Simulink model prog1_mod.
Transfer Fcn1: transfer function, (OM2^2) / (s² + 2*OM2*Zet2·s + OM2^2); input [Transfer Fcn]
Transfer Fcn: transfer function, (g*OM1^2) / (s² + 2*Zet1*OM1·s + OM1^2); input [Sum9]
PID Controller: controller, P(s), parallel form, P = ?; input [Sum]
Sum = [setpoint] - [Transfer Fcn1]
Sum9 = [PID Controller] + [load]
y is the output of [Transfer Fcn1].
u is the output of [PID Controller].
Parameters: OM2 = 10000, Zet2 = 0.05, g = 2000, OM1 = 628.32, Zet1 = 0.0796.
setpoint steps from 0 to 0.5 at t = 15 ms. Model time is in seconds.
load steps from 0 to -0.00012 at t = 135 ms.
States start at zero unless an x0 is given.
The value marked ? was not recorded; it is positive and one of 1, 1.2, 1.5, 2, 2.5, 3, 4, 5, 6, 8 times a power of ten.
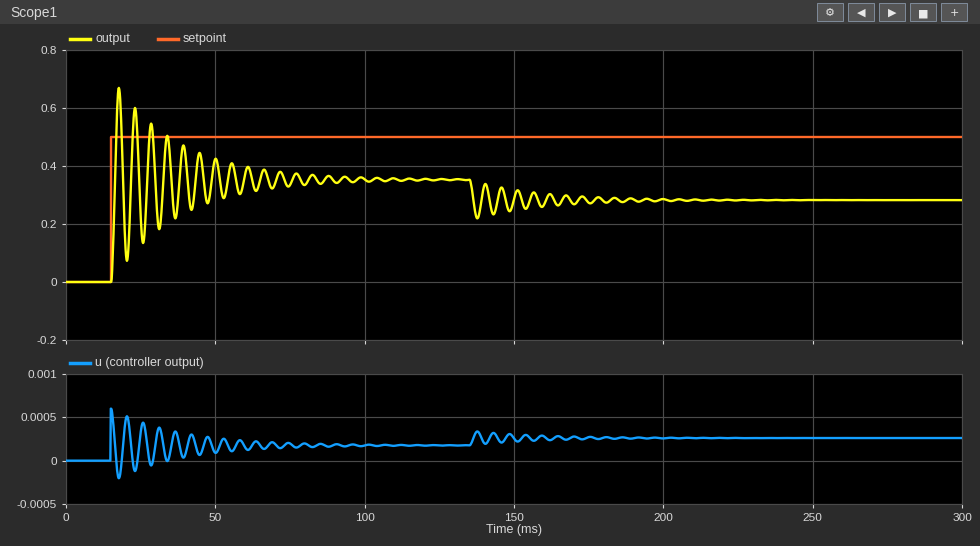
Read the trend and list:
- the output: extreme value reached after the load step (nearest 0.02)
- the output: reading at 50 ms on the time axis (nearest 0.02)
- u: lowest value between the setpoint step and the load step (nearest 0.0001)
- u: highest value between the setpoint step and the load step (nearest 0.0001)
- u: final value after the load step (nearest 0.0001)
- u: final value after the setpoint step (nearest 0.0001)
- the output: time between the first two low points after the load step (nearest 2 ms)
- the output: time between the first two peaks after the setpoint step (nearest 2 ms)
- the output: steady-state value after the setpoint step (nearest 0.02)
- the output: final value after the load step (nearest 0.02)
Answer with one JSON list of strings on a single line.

["0.22", "0.42", "-0.0002", "0.0006", "0.0003", "0.0002", "6 ms", "6 ms", "0.36", "0.28"]
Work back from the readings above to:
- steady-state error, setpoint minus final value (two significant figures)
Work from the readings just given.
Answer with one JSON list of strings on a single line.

["0.14"]
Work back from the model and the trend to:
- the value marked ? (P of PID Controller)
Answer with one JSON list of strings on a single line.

["0.0012"]
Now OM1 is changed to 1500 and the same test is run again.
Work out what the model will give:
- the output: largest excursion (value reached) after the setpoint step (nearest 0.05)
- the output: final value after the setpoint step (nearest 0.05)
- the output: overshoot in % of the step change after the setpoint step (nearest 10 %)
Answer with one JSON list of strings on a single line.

["0.70", "0.35", "100 %"]
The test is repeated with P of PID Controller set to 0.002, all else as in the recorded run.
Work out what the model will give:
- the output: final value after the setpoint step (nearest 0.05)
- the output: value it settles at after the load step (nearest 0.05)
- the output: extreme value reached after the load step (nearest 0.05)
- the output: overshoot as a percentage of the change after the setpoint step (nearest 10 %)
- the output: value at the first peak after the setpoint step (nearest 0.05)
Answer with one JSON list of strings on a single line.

["0.40", "0.35", "0.30", "90 %", "0.75"]
